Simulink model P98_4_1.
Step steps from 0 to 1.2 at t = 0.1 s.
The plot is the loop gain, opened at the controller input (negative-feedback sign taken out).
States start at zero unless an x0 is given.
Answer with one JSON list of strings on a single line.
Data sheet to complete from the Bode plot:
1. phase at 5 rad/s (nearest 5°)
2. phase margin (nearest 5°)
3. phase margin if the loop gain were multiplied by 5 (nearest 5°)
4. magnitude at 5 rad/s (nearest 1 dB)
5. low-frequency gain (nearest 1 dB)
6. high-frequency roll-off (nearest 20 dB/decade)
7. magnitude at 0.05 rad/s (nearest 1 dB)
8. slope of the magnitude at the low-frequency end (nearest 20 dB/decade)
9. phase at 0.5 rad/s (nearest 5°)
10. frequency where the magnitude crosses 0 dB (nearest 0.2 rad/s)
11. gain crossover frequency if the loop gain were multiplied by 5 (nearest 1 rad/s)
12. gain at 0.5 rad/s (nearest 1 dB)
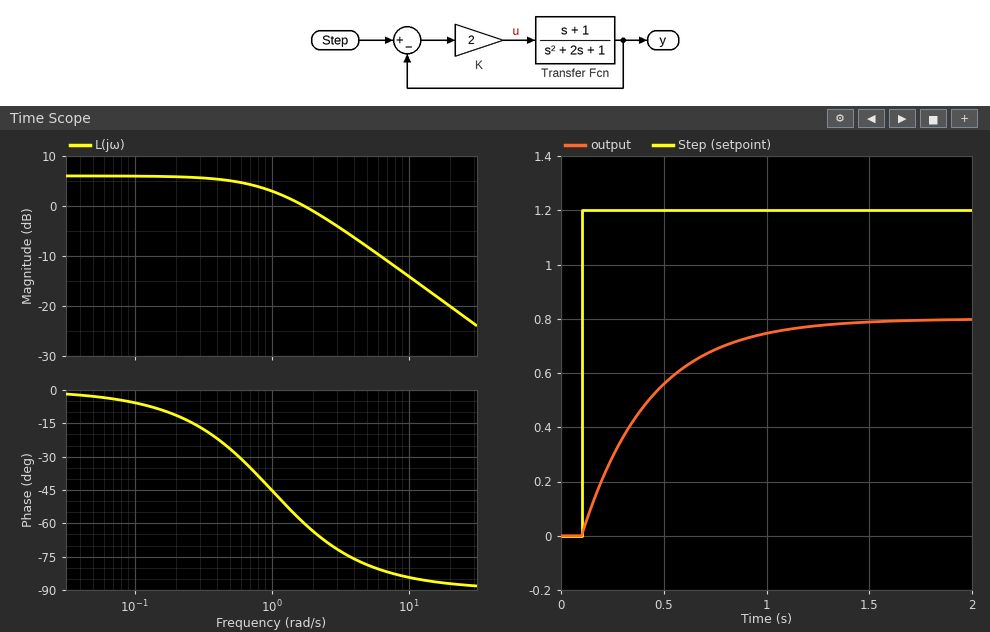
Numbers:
["-80°", "120°", "95°", "-8 dB", "6 dB", "-20 dB/decade", "6 dB", "0 dB/decade", "-25°", "1.8 rad/s", "10 rad/s", "5 dB"]
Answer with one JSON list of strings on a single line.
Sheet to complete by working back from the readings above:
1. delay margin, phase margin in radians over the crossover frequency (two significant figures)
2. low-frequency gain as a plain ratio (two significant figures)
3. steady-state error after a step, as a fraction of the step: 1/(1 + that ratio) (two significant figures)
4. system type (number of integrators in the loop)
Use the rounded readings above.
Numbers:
["1.2 s", "2.0", "0.33", "0"]
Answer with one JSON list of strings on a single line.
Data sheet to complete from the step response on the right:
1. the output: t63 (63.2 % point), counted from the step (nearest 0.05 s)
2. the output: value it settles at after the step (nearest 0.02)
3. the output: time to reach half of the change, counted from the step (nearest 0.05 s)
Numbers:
["0.35 s", "0.80", "0.25 s"]
